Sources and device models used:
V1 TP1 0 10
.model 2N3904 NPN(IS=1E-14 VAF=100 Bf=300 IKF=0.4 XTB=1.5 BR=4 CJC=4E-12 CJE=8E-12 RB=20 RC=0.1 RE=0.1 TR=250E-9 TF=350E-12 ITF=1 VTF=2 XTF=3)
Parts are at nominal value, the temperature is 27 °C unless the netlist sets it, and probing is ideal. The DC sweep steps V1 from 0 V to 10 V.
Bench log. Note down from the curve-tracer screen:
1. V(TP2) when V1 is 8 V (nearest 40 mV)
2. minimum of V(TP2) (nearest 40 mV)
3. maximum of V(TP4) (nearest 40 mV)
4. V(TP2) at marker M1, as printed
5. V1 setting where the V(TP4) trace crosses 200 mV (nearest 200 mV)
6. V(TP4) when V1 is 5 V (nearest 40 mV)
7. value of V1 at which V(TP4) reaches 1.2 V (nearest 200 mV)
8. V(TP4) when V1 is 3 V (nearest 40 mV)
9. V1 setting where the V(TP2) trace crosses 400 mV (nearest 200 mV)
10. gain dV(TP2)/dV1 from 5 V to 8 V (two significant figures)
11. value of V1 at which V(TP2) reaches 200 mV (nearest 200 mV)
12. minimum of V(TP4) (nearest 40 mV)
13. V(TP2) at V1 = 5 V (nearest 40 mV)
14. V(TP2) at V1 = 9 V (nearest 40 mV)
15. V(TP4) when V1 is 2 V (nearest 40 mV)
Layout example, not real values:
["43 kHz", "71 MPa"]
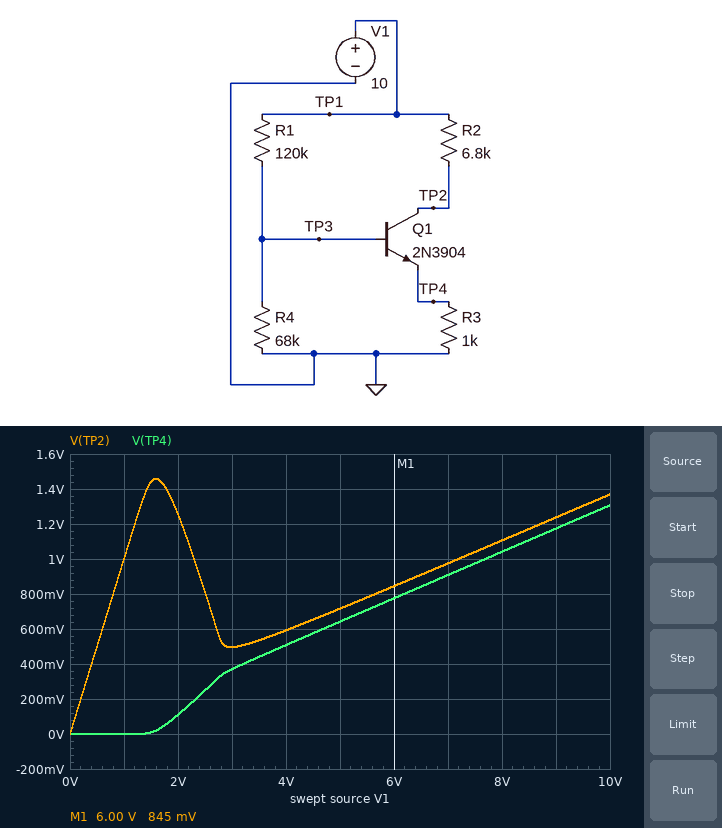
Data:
["1.12 V", "0 V", "1.32 V", "845 mV", "2.4 V", "640 mV", "9.2 V", "360 mV", "400 mV", "0.13 V/V", "200 mV", "0 V", "720 mV", "1.24 V", "120 mV"]
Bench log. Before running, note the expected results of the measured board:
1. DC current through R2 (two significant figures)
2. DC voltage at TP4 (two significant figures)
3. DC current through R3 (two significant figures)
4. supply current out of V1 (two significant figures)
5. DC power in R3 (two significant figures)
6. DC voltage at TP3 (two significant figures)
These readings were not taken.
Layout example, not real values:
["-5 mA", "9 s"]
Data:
["1.3 mA", "1.3 V", "1.3 mA", "1.3 mA", "1.7 mW", "2.0 V"]
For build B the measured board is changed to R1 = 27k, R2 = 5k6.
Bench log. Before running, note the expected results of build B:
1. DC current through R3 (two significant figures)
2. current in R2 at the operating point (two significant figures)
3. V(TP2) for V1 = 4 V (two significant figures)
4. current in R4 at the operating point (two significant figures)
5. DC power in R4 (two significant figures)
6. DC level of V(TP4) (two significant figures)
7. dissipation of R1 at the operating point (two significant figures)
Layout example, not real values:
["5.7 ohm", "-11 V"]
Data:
["1.7 mA", "1.5 mA", "700 mV", "35 µA", "85 µW", "1.7 V", "2.1 mW"]
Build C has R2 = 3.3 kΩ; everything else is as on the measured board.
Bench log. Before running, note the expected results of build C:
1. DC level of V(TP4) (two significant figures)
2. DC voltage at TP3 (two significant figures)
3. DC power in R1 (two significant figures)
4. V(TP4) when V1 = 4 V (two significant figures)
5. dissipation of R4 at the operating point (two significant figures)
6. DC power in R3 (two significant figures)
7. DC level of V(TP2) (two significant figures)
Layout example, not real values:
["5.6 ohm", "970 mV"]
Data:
["2.3 V", "3.0 V", "410 µW", "700 mV", "130 µW", "5.3 mW", "2.4 V"]
